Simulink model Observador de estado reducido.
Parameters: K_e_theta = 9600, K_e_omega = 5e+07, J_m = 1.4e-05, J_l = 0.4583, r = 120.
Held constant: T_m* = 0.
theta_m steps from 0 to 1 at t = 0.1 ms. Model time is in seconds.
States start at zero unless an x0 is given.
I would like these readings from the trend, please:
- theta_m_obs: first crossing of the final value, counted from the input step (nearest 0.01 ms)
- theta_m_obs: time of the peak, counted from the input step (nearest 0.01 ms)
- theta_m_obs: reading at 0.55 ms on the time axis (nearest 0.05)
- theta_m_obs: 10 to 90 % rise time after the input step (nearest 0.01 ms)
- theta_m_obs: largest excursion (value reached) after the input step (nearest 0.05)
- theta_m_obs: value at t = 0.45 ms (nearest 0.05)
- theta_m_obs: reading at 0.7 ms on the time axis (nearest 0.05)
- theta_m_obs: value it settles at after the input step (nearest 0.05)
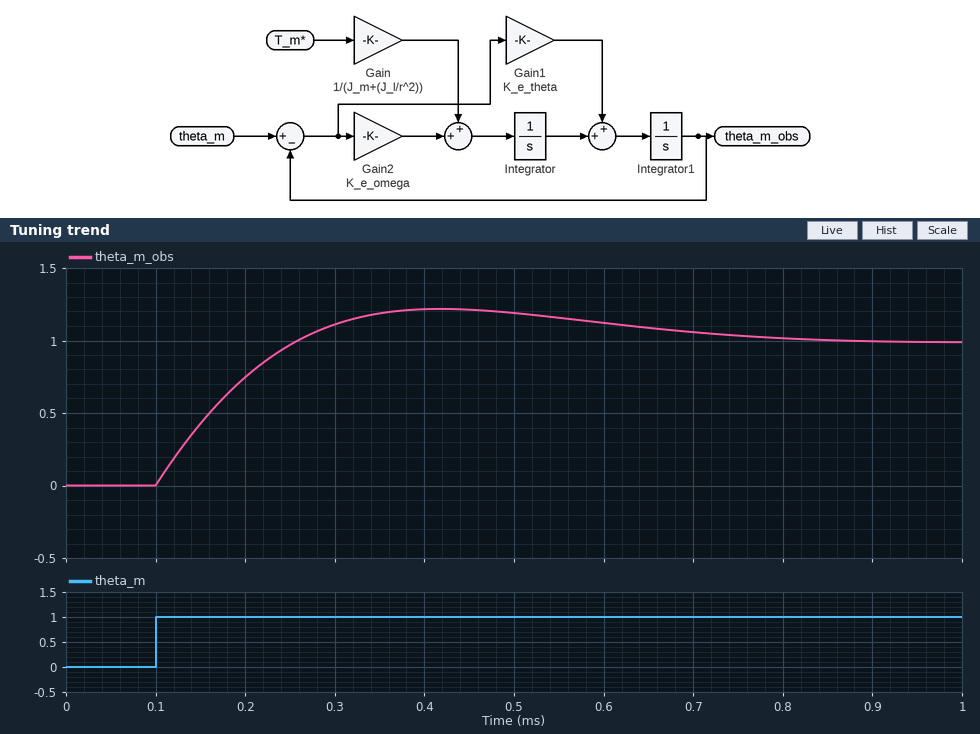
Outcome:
0.16 ms
0.32 ms
1.15
0.12 ms
1.20
1.20
1.05
1.00
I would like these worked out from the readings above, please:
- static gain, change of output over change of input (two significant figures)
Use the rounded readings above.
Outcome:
1.0
